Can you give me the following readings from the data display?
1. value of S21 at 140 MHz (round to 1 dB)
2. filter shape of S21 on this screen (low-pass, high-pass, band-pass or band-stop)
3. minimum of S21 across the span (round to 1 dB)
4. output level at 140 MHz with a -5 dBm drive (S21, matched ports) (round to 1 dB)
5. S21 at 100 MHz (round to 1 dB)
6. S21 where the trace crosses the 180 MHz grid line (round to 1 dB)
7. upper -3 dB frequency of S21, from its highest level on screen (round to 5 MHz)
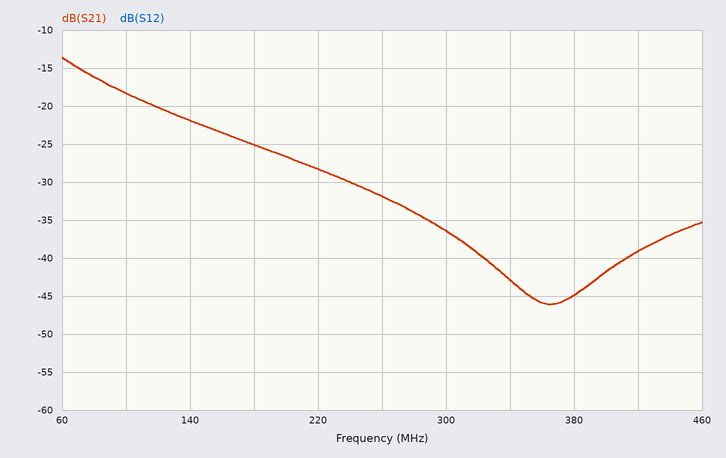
-22 dB
low-pass
-46 dB
-27 dBm
-18 dB
-25 dB
85 MHz
